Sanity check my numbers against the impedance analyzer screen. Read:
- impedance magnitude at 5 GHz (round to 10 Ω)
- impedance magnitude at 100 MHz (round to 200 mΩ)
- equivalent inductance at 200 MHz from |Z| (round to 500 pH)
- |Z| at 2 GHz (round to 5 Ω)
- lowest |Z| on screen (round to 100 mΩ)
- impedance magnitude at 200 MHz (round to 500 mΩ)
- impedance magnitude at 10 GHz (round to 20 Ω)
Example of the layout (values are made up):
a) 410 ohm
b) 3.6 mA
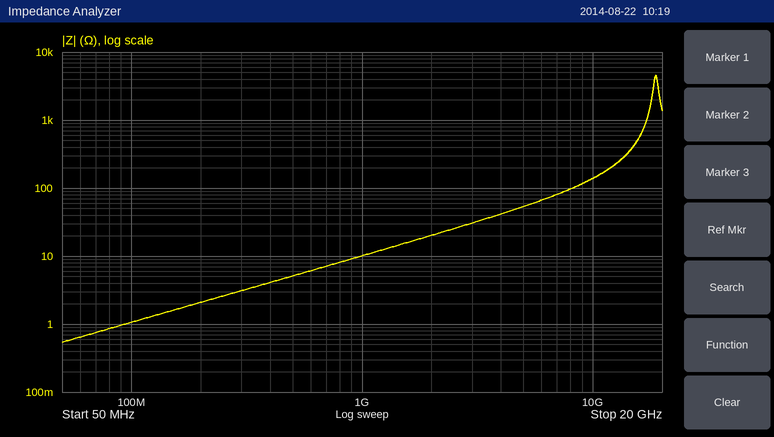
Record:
a) 50 Ω
b) 1.0 Ω
c) 1.5 nH
d) 20 Ω
e) 500 mΩ
f) 2.0 Ω
g) 140 Ω
